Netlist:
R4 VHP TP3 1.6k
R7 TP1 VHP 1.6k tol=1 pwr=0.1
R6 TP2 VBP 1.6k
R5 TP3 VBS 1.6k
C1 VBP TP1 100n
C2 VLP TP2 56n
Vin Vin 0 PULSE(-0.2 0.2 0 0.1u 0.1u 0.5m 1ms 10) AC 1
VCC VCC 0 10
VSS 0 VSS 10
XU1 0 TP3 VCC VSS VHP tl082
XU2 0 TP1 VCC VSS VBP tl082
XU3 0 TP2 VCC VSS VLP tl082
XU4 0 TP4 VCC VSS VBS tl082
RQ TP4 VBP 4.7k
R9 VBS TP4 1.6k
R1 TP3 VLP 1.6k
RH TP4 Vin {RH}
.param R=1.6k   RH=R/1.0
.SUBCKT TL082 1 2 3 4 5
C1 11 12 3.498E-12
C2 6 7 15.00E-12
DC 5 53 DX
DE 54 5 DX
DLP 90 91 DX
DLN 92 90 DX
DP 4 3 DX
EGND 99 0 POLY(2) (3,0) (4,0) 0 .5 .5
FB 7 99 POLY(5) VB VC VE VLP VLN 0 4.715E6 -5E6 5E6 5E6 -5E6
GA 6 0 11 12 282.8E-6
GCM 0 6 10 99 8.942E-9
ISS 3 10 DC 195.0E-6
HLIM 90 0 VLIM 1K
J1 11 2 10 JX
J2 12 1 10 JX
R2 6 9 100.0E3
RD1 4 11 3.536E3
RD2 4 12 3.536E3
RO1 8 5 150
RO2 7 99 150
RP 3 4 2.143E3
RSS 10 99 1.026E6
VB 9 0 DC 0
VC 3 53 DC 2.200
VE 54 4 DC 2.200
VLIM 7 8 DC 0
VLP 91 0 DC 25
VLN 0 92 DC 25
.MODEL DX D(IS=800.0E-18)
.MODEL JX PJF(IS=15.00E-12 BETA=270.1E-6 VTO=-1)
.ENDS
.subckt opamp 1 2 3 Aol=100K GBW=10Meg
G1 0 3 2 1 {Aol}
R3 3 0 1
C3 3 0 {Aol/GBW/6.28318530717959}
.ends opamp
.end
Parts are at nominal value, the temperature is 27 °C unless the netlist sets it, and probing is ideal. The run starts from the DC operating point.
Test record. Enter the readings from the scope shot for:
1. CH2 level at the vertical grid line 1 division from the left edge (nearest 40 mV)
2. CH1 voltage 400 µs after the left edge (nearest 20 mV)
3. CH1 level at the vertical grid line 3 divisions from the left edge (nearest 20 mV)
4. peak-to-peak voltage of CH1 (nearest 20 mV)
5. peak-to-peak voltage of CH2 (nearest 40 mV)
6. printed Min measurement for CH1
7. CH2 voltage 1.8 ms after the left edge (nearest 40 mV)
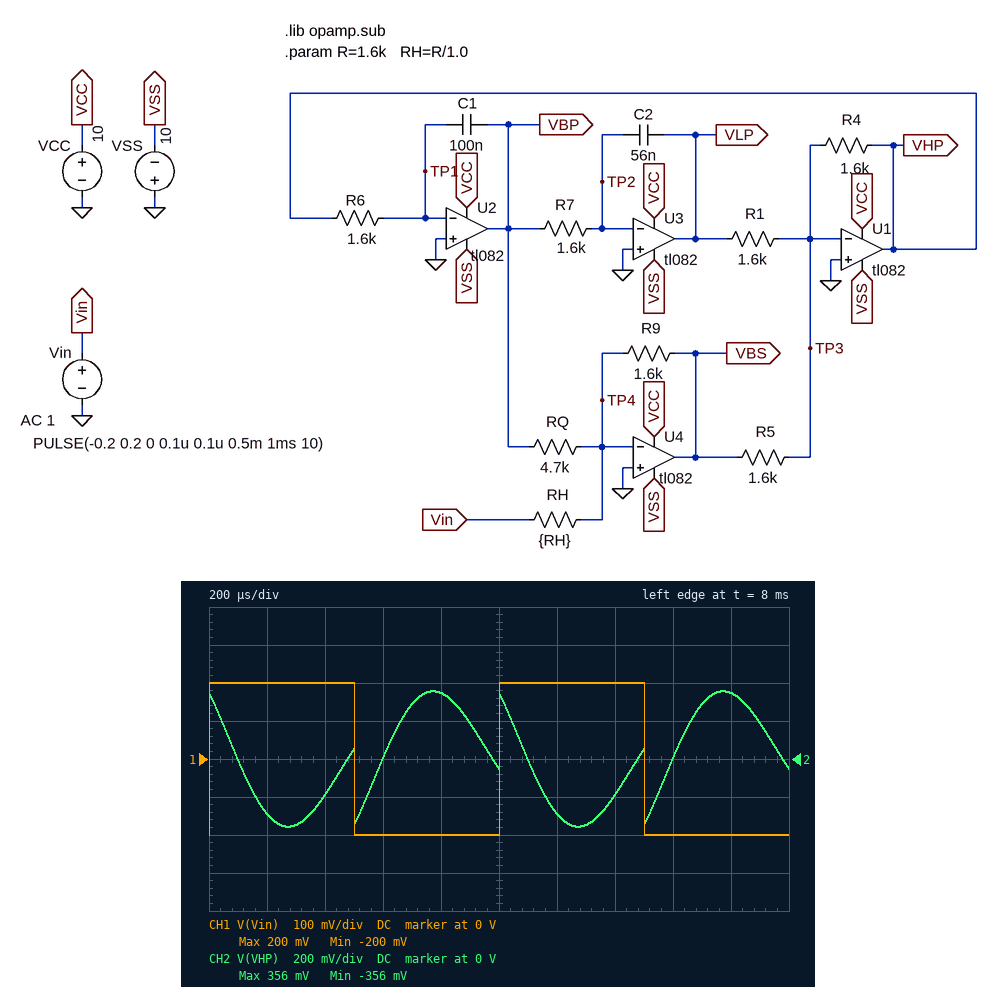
-280 mV
200 mV
-200 mV
400 mV
720 mV
-200 mV
360 mV
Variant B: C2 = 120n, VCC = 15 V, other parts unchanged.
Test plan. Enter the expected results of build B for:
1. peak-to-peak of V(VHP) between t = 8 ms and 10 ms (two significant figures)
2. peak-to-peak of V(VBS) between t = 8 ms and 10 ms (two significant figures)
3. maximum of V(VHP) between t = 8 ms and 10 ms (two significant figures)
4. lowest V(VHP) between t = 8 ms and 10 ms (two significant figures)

1.6 V
650 mV
820 mV
-820 mV
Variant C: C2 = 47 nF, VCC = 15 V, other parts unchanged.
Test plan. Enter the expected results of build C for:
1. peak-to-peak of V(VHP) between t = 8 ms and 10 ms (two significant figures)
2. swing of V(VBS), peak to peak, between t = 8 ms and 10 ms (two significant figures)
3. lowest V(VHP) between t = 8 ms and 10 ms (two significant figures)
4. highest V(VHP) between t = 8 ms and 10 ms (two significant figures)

580 mV
510 mV
-290 mV
290 mV
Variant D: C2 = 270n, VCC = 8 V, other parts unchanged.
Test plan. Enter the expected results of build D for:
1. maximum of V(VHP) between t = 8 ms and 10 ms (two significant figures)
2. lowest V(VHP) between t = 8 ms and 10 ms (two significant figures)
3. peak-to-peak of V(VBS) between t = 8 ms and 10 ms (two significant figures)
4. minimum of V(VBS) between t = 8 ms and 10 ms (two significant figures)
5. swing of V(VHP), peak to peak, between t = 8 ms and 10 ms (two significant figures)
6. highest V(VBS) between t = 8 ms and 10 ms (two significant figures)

390 mV
-390 mV
650 mV
-330 mV
780 mV
330 mV
